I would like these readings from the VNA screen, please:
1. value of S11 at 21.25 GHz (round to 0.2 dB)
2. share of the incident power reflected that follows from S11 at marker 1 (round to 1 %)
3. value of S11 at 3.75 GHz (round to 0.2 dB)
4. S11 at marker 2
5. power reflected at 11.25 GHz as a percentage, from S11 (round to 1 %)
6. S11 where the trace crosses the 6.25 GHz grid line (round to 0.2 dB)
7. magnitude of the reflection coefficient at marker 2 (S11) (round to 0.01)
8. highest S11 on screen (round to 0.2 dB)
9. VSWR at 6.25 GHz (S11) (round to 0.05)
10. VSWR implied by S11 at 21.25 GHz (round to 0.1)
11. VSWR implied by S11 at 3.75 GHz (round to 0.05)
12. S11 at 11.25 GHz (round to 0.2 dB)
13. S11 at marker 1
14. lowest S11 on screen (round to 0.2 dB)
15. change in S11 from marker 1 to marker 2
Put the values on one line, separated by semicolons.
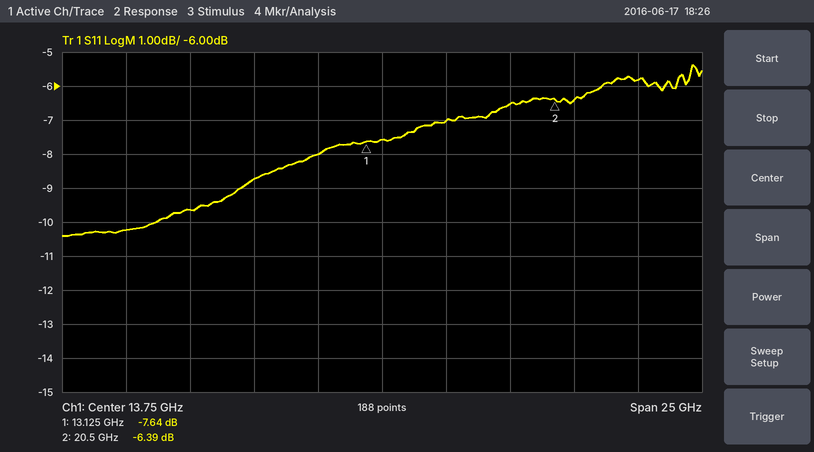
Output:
-6.4 dB; 17 %; -10.2 dB; -6.39 dB; 16 %; -9.6 dB; 0.48; -5.4 dB; 2.00; 2.8; 1.90; -8.0 dB; -7.64 dB; -10.4 dB; 1.25 dB
